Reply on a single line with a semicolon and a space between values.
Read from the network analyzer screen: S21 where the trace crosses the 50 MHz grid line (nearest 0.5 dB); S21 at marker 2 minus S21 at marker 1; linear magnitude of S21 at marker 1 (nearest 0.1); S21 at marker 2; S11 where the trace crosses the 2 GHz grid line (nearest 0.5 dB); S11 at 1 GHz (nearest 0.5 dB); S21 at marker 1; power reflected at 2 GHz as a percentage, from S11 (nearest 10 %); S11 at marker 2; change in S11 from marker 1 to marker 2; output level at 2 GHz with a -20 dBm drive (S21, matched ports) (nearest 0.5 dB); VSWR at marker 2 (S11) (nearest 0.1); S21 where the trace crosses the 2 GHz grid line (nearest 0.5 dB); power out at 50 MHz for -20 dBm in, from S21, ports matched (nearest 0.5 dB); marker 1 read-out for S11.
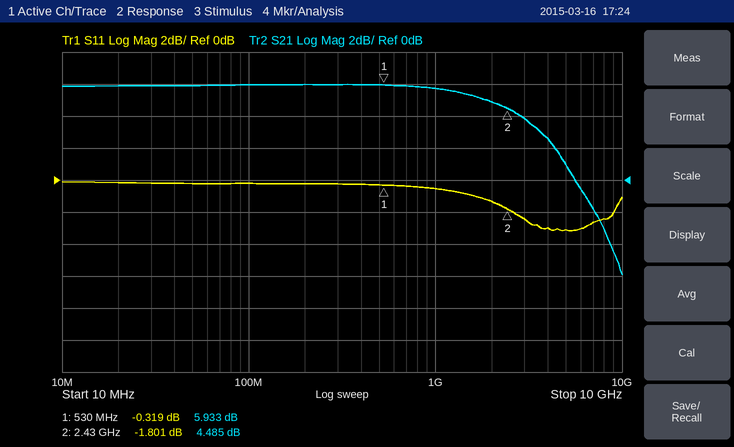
6.0 dB; -1.448 dB; 2.0; 4.485 dB; -1.5 dB; -0.5 dB; 5.933 dB; 70 %; -1.801 dB; -1.482 dB; -15.0 dBm; 9.7; 5.0 dB; -14.0 dBm; -0.319 dB
